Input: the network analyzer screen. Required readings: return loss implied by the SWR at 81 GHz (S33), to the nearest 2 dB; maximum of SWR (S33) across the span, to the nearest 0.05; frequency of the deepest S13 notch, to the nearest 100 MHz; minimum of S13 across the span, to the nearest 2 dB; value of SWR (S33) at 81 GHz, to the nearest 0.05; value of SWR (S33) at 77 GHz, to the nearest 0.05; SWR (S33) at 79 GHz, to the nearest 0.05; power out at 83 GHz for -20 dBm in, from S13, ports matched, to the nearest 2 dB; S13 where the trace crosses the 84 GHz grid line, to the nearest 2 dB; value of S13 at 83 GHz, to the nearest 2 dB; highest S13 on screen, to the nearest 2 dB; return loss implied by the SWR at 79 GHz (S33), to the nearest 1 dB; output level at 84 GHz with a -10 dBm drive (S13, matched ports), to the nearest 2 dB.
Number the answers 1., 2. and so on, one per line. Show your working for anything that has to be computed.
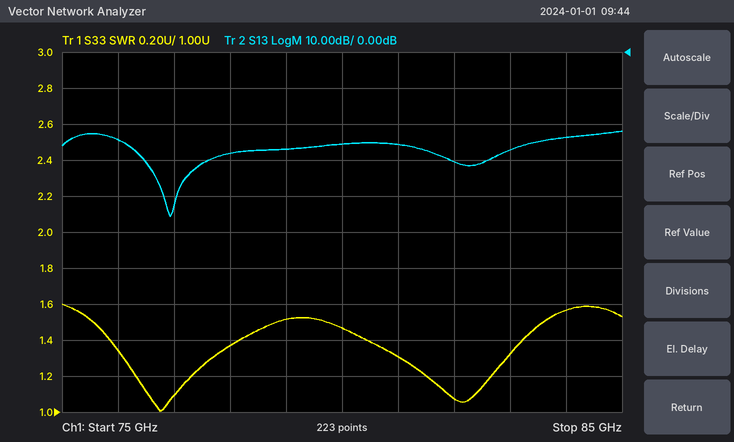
1. −20 log10((1.3 − 1)/(1.3 + 1)) ≈ 18 dB
2. 1.60
3. 76.9 GHz
4. -46 dB
5. 1.30
6. 1.10
7. 1.50
8. -20 dBm + (-28 dB) = -48 dBm
9. -24 dB
10. -28 dB
11. -22 dB
12. −20 log10((1.5 − 1)/(1.5 + 1)) ≈ 14 dB
13. -10 dBm + (-24 dB) = -34 dBm
